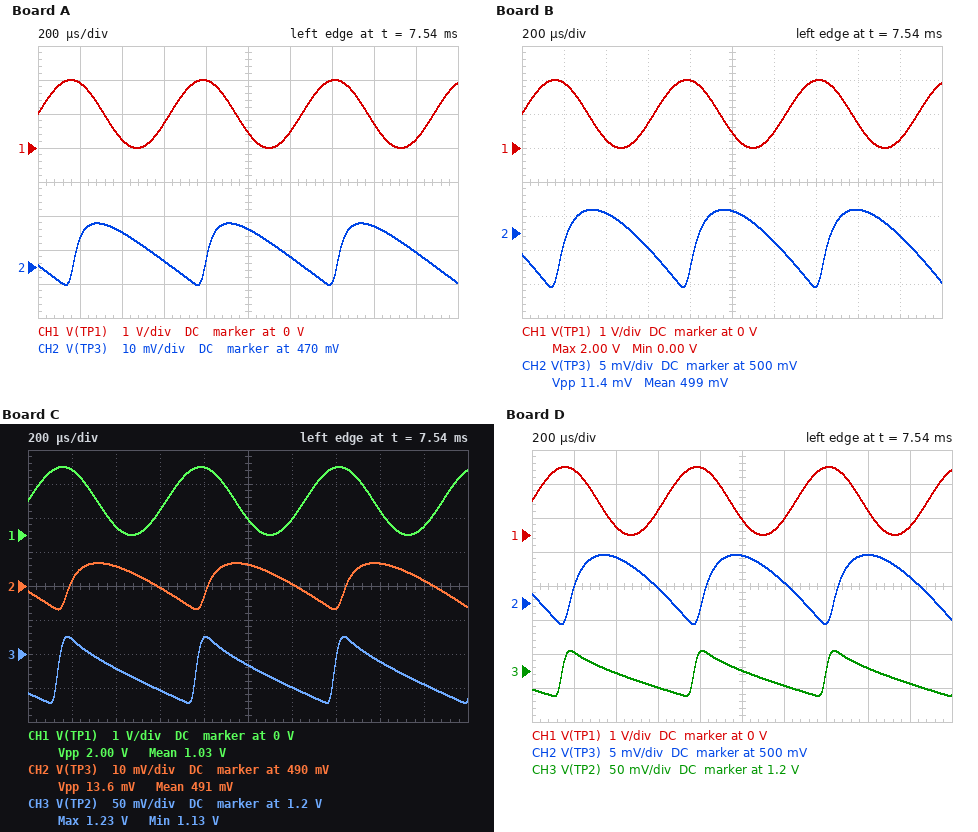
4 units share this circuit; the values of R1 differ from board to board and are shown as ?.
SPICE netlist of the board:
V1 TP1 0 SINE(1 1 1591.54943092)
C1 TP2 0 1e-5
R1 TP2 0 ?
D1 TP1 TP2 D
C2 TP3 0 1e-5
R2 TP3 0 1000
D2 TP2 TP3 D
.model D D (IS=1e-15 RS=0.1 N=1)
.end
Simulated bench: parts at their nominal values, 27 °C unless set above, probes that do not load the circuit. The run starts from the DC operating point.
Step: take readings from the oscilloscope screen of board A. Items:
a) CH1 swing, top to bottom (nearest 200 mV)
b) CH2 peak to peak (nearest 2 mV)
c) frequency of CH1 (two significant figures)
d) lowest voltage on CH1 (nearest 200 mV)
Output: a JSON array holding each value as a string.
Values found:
["2.0 V", "18 mV", "1.6 kHz", "0 V"]
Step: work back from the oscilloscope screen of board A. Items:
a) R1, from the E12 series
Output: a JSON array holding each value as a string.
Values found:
["390 Ω"]
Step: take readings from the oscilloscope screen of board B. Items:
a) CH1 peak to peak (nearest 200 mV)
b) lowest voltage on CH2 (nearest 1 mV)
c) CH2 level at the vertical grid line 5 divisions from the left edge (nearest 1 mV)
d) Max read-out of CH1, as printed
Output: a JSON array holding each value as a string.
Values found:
["2.0 V", "492 mV", "503 mV", "2.00 V"]
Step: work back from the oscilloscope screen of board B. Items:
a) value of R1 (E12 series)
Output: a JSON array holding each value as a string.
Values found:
["1.2 kΩ"]
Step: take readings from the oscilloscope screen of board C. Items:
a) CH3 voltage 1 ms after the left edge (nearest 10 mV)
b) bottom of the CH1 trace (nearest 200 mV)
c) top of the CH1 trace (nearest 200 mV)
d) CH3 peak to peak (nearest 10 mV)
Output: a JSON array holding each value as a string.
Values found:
["1.18 V", "0 V", "2.0 V", "100 mV"]
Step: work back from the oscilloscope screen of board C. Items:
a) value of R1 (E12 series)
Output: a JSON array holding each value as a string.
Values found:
["820 Ω"]
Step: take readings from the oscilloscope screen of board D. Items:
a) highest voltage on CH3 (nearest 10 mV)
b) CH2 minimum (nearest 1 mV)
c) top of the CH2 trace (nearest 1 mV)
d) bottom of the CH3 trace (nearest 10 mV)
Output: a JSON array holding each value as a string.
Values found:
["1.23 V", "497 mV", "507 mV", "1.16 V"]
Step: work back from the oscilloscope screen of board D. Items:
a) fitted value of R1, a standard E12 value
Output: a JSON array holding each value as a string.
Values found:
["1.5 kΩ"]
